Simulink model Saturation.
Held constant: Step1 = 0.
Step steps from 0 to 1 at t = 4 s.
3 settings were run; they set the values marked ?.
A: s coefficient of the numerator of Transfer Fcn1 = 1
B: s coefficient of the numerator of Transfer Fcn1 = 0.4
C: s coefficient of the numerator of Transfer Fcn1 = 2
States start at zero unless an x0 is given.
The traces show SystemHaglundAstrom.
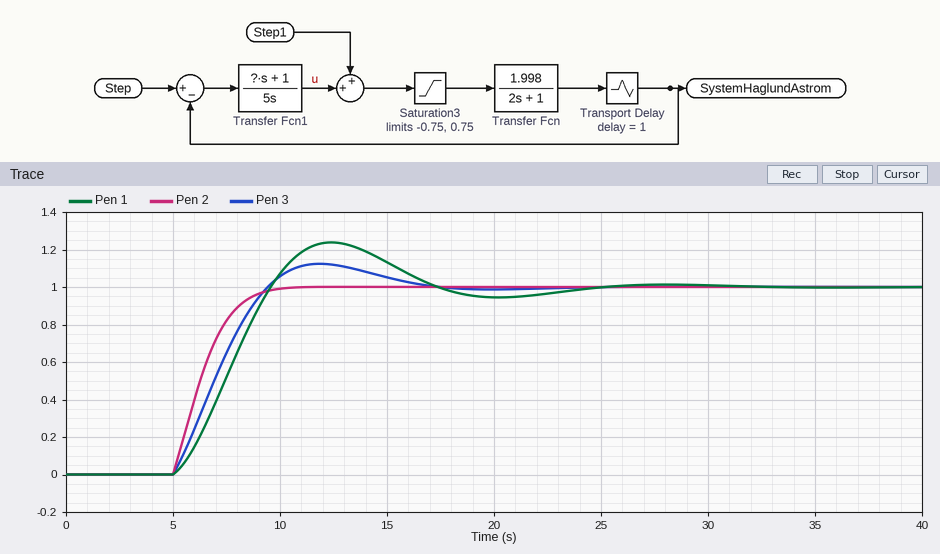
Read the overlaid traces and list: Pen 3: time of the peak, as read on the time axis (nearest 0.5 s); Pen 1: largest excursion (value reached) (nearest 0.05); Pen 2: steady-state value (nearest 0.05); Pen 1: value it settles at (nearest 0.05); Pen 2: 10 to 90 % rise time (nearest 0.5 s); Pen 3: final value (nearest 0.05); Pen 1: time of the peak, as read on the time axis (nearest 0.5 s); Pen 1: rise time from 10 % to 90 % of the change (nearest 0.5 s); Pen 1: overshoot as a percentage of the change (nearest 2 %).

12.0 s
1.25
1.00
1.00
3.0 s
1.00
12.5 s
3.5 s
24 %
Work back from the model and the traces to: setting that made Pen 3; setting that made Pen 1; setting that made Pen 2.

A
B
C
